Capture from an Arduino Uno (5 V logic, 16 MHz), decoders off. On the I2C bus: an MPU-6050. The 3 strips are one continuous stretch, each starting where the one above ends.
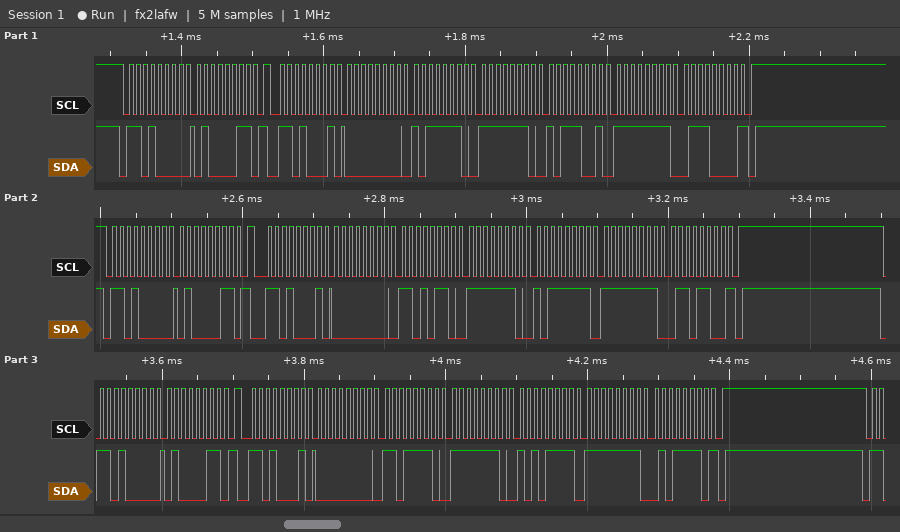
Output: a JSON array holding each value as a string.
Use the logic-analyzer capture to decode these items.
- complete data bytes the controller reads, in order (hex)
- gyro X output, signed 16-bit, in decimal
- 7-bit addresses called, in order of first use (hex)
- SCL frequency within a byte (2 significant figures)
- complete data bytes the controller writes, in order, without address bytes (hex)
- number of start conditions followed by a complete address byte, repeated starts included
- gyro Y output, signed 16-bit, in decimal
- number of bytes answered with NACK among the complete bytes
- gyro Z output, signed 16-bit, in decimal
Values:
["00 BE FE B9 FF 70 00 D6 FE BF FF 6C 00 DE FE AF FF 5E", "190", "0x68", "100 kHz", "43 43 43", "6", "-327", "3", "-144"]
